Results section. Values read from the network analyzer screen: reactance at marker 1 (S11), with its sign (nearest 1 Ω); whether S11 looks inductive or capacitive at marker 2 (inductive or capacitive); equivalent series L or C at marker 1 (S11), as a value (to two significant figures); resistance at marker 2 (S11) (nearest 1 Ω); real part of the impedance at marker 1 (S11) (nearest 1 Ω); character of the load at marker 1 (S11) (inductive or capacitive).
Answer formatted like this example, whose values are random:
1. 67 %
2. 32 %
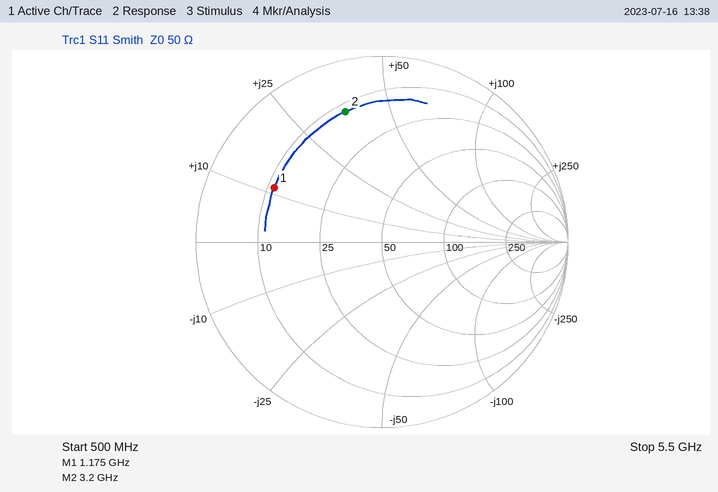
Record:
1. +11 Ω
2. inductive
3. 1.5 nH
4. 12 Ω
5. 11 Ω
6. inductive
